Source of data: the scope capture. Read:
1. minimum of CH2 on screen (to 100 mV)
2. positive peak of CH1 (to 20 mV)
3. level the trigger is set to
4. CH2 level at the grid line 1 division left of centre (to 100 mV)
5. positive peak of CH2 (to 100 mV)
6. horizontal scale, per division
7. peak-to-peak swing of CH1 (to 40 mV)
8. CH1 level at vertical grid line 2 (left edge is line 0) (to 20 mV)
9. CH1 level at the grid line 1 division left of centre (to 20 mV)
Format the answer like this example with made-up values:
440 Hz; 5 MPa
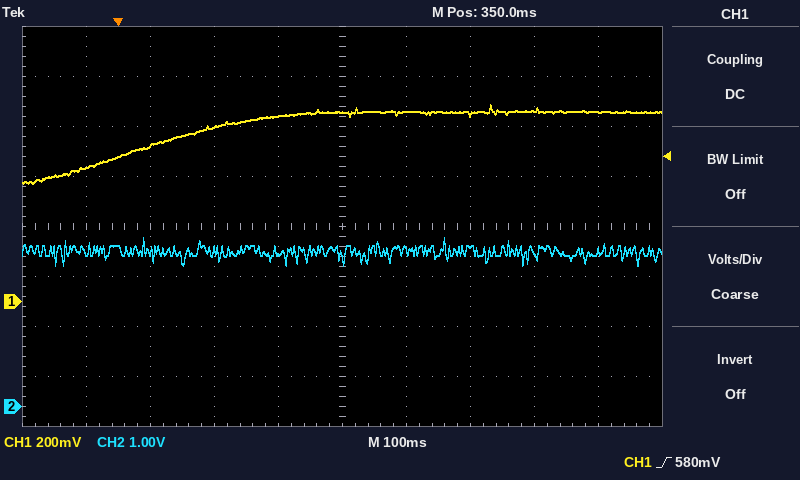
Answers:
2.8 V; 780 mV; 580 mV; 3.1 V; 3.4 V; 100 ms; 320 mV; 620 mV; 740 mV
